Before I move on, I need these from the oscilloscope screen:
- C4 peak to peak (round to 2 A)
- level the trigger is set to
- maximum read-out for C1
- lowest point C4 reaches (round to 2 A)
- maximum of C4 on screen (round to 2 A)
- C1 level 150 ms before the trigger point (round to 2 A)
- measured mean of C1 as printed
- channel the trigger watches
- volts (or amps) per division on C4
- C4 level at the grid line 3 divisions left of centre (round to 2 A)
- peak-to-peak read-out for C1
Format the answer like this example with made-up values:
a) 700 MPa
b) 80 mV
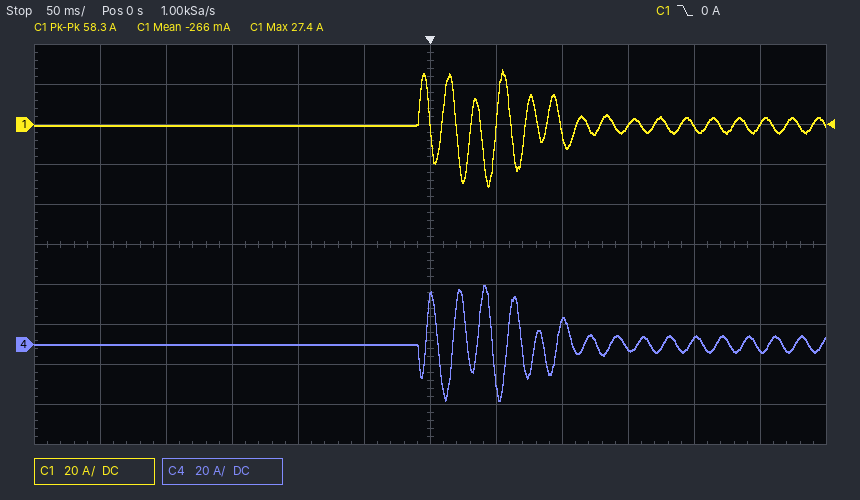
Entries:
a) 58 A
b) 0 A
c) 27.4 A
d) -28 A
e) 30 A
f) 0 A
g) -266 mA
h) C1
i) 20 A
j) 0 A
k) 58.3 A
